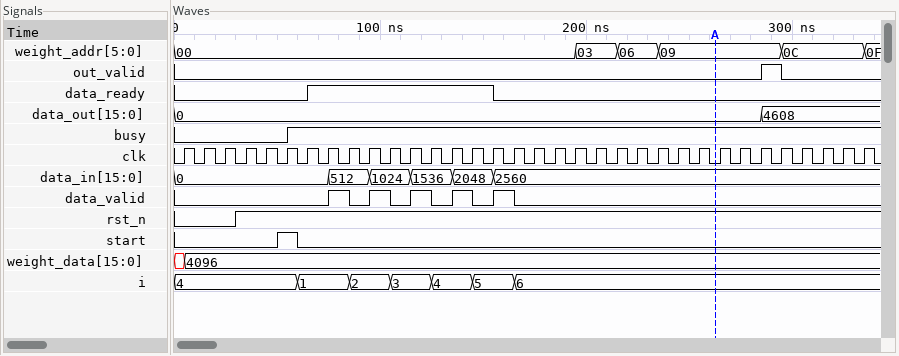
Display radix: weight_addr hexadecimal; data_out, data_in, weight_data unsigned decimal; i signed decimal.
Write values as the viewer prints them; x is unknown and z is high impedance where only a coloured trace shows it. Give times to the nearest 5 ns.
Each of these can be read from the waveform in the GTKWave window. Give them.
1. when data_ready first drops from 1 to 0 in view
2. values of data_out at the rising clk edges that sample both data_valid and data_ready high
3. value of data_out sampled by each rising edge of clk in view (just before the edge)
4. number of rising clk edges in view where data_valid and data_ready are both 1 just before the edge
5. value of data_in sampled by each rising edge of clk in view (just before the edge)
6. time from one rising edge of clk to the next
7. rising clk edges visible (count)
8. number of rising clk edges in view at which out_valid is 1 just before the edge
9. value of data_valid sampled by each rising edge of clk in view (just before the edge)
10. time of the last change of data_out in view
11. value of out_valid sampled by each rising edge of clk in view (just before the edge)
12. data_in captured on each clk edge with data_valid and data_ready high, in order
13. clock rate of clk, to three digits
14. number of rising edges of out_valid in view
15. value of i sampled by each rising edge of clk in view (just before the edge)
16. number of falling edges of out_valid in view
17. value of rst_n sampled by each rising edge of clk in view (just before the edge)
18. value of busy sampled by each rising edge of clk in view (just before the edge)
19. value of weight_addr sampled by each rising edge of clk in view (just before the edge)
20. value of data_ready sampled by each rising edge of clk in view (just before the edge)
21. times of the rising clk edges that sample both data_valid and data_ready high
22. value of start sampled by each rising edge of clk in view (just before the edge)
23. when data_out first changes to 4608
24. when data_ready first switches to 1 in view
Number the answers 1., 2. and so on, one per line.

1. 155 ns
2. 0, 0, 0, 0
3. 0, 0, 0, 0, 0, 0, 0, 0, 0, 0, 0, 0, 0, 0, 0, 0, 0, 0, 0, 0, 0, 0, 0, 0, 0, 0, 0, 0, 0, 4608, 4608, 4608, 4608, 4608
4. 4
5. 0, 0, 0, 0, 0, 0, 0, 0, 512, 512, 1024, 1024, 1536, 1536, 2048, 2048, 2560, 2560, 2560, 2560, 2560, 2560, 2560, 2560, 2560, 2560, 2560, 2560, 2560, 2560, 2560, 2560, 2560, 2560
6. 10 ns
7. 34
8. 1
9. 0 0 0 0 0 0 0 0 1 0 1 0 1 0 1 0 1 0 0 0 0 0 0 0 0 0 0 0 0 0 0 0 0 0
10. 285 ns
11. 0 0 0 0 0 0 0 0 0 0 0 0 0 0 0 0 0 0 0 0 0 0 0 0 0 0 0 0 0 1 0 0 0 0
12. 512, 1024, 1536, 2048
13. 100 MHz
14. 1
15. 4, 4, 4, 4, 4, 4, 1, 1, 1, 2, 2, 3, 3, 4, 4, 5, 5, 6, 6, 6, 6, 6, 6, 6, 6, 6, 6, 6, 6, 6, 6, 6, 6, 6
16. 1
17. 0 0 0 1 1 1 1 1 1 1 1 1 1 1 1 1 1 1 1 1 1 1 1 1 1 1 1 1 1 1 1 1 1 1
18. 0 0 0 0 0 0 1 1 1 1 1 1 1 1 1 1 1 1 1 1 1 1 1 1 1 1 1 1 1 1 1 1 1 1
19. 00, 00, 00, 00, 00, 00, 00, 00, 00, 00, 00, 00, 00, 00, 00, 00, 00, 00, 00, 00, 03, 03, 06, 06, 09, 09, 09, 09, 09, 09, 0C, 0C, 0C, 0C
20. 0 0 0 0 0 0 0 1 1 1 1 1 1 1 1 1 0 0 0 0 0 0 0 0 0 0 0 0 0 0 0 0 0 0
21. 85 ns, 105 ns, 125 ns, 145 ns
22. 0 0 0 0 0 1 0 0 0 0 0 0 0 0 0 0 0 0 0 0 0 0 0 0 0 0 0 0 0 0 0 0 0 0
23. 285 ns
24. 65 ns
